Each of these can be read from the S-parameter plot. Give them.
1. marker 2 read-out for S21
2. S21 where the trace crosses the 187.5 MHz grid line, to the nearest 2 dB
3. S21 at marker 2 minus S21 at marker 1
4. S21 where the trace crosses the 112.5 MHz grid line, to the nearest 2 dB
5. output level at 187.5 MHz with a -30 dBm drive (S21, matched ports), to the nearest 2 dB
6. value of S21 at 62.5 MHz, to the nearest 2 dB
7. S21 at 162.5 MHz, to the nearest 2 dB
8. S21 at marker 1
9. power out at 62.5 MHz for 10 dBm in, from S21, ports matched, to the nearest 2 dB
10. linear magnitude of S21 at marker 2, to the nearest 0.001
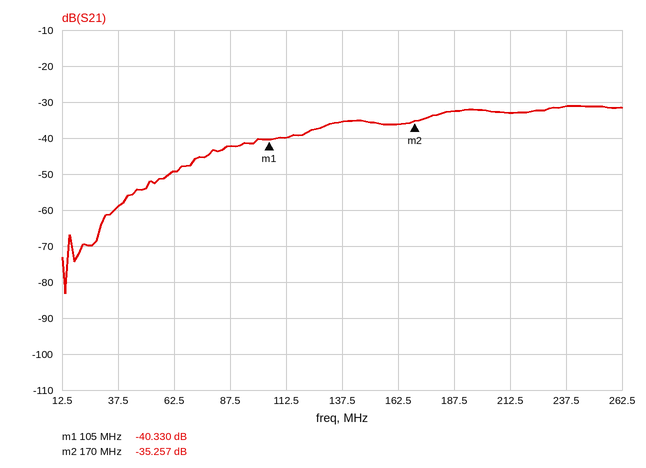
-35.257 dB
-32 dB
5.073 dB
-40 dB
-62 dBm
-50 dB
-36 dB
-40.330 dB
-40 dBm
0.017
